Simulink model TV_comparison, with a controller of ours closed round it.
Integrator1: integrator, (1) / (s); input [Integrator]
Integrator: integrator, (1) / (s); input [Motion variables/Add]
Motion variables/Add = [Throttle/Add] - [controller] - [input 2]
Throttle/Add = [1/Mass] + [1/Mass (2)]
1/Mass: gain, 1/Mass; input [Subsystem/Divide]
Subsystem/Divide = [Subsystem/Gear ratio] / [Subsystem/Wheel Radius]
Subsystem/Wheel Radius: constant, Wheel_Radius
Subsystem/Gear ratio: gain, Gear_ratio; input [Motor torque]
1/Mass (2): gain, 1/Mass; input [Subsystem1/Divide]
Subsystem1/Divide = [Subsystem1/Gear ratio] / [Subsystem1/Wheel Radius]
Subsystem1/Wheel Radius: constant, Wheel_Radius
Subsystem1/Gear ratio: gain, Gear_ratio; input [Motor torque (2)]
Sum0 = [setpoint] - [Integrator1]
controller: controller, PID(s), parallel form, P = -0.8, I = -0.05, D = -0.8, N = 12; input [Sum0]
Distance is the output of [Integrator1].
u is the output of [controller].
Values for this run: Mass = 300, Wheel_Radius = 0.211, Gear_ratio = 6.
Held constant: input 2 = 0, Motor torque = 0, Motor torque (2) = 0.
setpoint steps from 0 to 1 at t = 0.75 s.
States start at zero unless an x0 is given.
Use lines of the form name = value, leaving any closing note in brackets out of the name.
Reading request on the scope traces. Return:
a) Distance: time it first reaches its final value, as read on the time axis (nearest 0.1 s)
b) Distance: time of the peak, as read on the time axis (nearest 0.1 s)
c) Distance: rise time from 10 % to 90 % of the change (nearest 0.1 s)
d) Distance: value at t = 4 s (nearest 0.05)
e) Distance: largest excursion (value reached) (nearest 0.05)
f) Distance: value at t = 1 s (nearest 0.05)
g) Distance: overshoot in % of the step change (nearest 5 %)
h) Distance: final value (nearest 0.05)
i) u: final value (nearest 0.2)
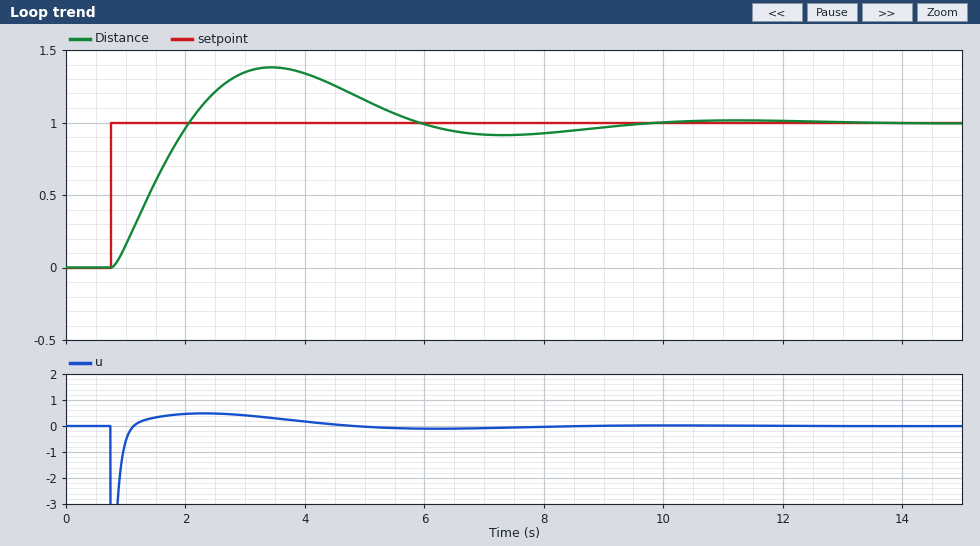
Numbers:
Distance: time it first reaches its final value, as read on the time axis = 2.1 s
Distance: time of the peak, as read on the time axis = 3.4 s
Distance: rise time from 10 % to 90 % of the change = 1.0 s
Distance: value at t = 4 s = 1.35
Distance: largest excursion (value reached) = 1.40
Distance: value at t = 1 s = 0.15
Distance: overshoot in % of the step change = 40 %
Distance: final value = 1.00
u: final value = 0.0
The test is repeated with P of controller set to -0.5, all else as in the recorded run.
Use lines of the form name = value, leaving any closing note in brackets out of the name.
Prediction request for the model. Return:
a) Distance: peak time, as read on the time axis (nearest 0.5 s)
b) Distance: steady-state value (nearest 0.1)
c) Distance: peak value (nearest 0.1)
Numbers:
Distance: peak time, as read on the time axis = 4.0 s
Distance: steady-state value = 1.0
Distance: peak value = 1.3
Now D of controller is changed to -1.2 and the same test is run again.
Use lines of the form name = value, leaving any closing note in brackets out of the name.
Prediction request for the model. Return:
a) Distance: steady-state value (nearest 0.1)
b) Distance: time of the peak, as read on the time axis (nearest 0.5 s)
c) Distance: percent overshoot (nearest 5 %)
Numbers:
Distance: steady-state value = 1.0
Distance: time of the peak, as read on the time axis = 3.0 s
Distance: percent overshoot = 25 %
